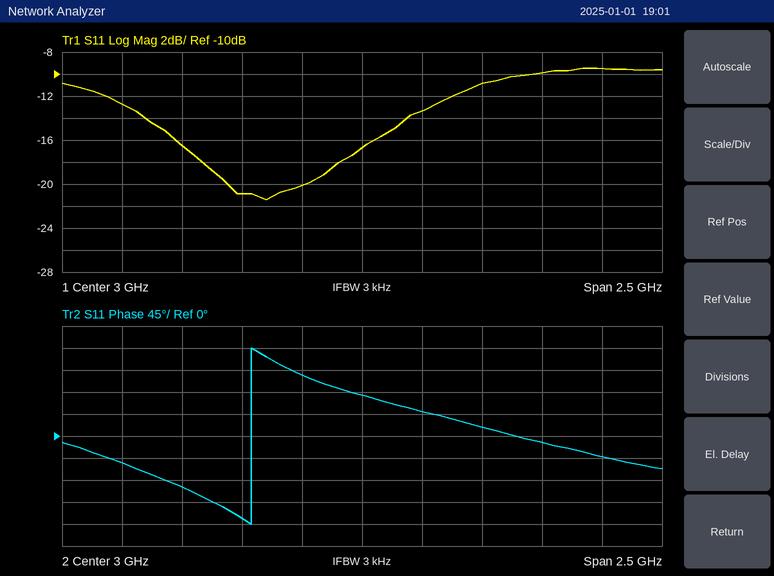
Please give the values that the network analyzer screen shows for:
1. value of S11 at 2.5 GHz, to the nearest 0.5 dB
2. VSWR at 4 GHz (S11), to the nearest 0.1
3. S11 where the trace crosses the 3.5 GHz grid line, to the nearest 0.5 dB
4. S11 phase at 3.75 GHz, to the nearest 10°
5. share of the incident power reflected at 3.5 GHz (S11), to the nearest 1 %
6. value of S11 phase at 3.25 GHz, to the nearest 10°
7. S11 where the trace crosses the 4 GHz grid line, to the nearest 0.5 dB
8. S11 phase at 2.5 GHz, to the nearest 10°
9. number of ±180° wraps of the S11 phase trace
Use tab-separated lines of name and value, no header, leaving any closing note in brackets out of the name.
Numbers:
value of S11 at 2.5 GHz, to the nearest 0.5 dB	-21.0 dB
VSWR at 4 GHz (S11), to the nearest 0.1	2.0
S11 where the trace crosses the 3.5 GHz grid line, to the nearest 0.5 dB	-11.0 dB
S11 phase at 3.75 GHz, to the nearest 10°	-10°
share of the incident power reflected at 3.5 GHz (S11), to the nearest 1 %	8 %
value of S11 phase at 3.25 GHz, to the nearest 10°	50°
S11 where the trace crosses the 4 GHz grid line, to the nearest 0.5 dB	-9.5 dB
S11 phase at 2.5 GHz, to the nearest 10°	-170°
number of ±180° wraps of the S11 phase trace	1
